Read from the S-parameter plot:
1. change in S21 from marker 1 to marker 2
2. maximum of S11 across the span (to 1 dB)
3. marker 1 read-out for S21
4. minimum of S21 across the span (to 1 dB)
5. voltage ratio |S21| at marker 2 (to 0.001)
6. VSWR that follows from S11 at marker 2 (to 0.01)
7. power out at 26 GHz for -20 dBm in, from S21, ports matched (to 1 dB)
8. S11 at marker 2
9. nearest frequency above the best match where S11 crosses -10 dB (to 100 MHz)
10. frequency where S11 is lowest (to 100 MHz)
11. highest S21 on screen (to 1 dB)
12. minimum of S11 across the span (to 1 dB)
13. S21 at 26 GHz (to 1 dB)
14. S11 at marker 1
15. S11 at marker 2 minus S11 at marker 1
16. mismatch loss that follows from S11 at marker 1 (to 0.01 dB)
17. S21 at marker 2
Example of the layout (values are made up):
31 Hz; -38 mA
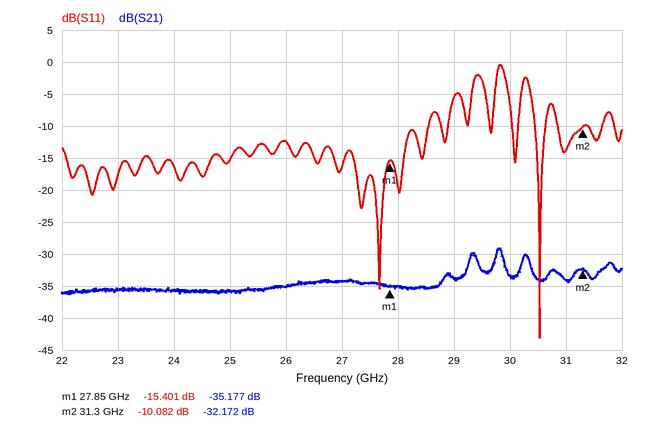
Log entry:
3.005 dB; 0 dB; -35.177 dB; -36 dB; 0.025; 1.91; -55 dBm; -10.082 dB; 30.6 GHz; 30.5 GHz; -29 dB; -43 dB; -35 dB; -15.401 dB; 5.319 dB; 0.13 dB; -32.172 dB
